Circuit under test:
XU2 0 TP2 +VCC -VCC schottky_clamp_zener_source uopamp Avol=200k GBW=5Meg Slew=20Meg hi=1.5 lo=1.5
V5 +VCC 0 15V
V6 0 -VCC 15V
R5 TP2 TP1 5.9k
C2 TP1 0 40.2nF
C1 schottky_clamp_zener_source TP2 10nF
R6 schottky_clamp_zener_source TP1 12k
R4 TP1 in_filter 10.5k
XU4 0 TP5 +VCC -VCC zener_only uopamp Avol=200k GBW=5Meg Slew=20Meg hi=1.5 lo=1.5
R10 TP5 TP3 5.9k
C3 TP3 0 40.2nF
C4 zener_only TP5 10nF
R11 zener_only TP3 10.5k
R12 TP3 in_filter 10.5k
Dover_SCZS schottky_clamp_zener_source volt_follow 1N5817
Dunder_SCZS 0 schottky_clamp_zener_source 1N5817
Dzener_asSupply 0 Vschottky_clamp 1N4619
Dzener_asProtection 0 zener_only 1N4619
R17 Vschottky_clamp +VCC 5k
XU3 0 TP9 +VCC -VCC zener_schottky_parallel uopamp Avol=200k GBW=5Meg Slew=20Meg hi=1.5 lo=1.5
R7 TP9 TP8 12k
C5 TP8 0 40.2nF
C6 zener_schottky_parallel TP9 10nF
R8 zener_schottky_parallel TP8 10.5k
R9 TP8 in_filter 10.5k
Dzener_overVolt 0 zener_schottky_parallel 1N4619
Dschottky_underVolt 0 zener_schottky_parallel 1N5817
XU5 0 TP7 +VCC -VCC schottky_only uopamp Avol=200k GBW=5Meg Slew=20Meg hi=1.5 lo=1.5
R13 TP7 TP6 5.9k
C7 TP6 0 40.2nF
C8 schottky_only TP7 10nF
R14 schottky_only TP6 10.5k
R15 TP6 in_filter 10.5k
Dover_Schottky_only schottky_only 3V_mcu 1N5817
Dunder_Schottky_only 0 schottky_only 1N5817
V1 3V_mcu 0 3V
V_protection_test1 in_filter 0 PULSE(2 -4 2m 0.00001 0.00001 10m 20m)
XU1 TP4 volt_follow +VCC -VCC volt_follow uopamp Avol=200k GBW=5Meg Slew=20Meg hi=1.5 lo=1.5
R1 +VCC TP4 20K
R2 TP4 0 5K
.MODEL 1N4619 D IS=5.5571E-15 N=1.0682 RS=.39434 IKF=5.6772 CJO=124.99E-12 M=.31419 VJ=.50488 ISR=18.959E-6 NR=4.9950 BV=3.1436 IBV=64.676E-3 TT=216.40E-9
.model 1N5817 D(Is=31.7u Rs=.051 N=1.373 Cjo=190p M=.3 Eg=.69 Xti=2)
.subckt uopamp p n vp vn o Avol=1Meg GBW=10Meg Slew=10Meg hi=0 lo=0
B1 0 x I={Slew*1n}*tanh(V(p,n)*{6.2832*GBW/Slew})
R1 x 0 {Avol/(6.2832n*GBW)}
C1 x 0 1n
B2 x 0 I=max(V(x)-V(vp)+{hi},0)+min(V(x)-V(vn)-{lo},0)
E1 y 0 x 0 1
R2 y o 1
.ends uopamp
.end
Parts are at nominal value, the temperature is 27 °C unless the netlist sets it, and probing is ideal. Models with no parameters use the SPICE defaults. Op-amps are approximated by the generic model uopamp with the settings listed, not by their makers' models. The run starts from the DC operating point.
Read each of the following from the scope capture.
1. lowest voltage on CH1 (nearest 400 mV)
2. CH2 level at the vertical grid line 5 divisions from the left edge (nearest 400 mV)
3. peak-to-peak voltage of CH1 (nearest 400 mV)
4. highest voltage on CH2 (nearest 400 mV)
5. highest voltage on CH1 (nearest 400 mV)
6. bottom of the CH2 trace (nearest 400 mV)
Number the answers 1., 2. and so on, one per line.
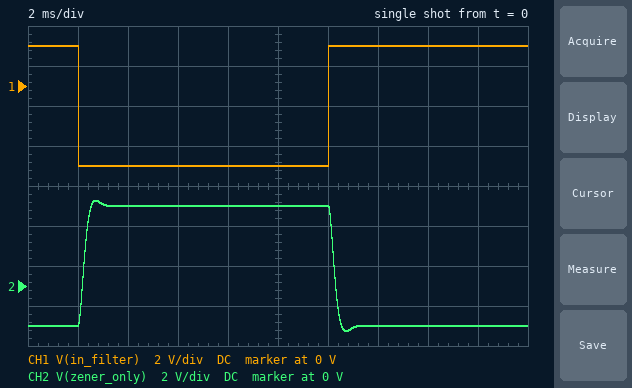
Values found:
1. -4.0 V
2. 4.0 V
3. 6.0 V
4. 4.4 V
5. 2.0 V
6. -2.4 V
